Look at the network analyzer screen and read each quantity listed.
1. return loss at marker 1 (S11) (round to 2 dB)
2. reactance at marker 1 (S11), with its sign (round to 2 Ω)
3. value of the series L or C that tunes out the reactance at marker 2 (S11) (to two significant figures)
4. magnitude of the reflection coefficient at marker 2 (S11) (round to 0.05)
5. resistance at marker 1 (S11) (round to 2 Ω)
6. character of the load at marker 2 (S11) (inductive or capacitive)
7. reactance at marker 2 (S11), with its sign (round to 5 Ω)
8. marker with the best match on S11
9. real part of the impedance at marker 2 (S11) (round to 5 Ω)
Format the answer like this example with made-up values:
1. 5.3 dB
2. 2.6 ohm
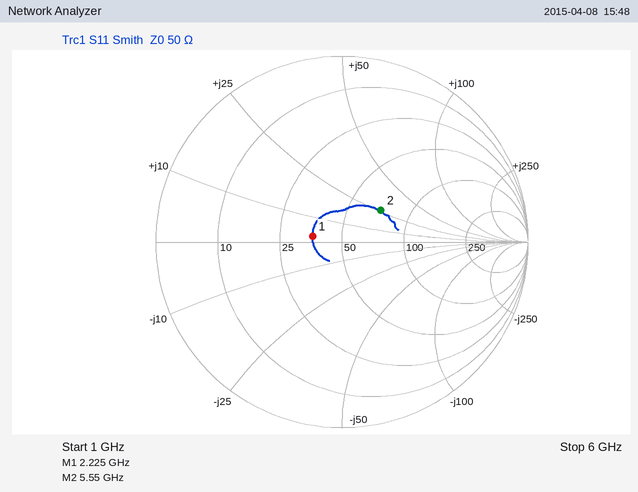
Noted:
1. 16 dB
2. +2 Ω
3. 1.1 pF
4. 0.25
5. 36 Ω
6. inductive
7. +25 Ω
8. marker 1
9. 70 Ω
